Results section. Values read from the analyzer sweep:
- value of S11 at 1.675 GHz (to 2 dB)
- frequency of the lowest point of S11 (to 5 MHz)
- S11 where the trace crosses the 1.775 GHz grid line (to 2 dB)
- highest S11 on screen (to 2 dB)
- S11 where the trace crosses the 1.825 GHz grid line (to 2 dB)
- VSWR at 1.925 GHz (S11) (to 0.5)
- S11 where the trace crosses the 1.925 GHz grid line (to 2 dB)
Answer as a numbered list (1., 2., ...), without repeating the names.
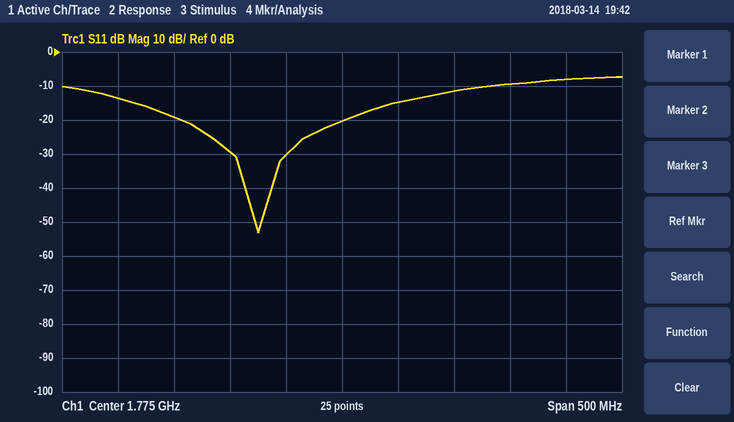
1. -30 dB
2. 1.700 GHz
3. -20 dB
4. -8 dB
5. -14 dB
6. 2.0
7. -10 dB
